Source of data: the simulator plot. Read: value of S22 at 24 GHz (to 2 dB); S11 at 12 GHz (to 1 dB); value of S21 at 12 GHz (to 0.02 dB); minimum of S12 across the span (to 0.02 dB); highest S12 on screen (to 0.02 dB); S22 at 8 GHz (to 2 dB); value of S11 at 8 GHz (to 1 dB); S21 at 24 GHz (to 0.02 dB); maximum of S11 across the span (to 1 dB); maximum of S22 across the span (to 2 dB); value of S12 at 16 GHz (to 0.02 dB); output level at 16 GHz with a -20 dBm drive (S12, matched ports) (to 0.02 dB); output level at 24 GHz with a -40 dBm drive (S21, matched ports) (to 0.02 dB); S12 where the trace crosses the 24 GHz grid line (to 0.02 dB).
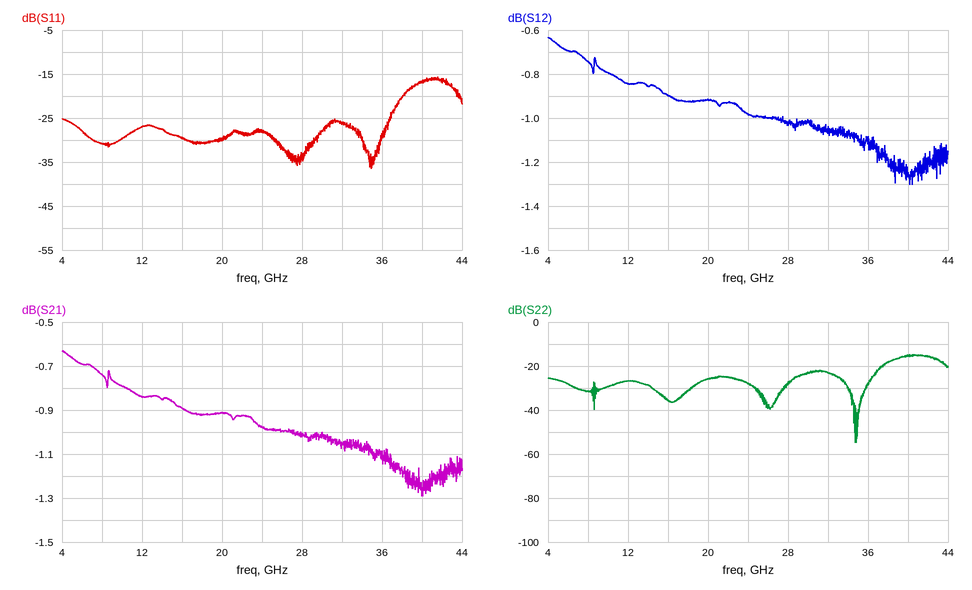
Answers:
-28 dB
-27 dB
-0.84 dB
-1.30 dB
-0.64 dB
-32 dB
-31 dB
-0.98 dB
-16 dB
-14 dB
-0.90 dB
-20.90 dBm
-40.98 dBm
-0.98 dB
